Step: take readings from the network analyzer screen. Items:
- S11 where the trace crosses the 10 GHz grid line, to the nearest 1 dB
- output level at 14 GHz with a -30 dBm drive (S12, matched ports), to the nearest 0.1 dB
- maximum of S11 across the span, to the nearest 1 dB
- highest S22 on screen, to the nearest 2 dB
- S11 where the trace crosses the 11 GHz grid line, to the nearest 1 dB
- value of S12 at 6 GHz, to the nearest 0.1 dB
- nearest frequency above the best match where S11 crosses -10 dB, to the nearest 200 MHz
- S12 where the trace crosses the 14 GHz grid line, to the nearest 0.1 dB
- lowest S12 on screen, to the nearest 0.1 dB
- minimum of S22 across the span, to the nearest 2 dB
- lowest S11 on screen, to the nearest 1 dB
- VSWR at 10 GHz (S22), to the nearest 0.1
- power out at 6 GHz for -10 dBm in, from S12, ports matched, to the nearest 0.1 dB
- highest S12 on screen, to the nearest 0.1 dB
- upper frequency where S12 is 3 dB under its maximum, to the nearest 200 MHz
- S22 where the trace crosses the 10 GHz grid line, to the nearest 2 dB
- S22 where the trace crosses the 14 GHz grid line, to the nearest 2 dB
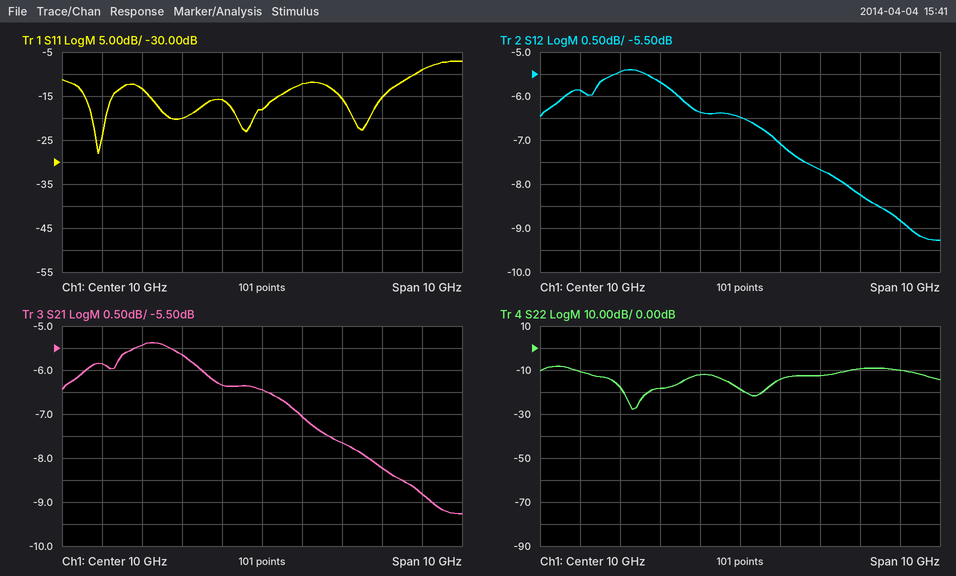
-18 dB
-38.8 dBm
-7 dB
-8 dB
-12 dB
-5.9 dB
13.8 GHz
-8.8 dB
-9.3 dB
-28 dB
-28 dB
1.3
-15.9 dBm
-5.4 dB
13.2 GHz
-18 dB
-10 dB
